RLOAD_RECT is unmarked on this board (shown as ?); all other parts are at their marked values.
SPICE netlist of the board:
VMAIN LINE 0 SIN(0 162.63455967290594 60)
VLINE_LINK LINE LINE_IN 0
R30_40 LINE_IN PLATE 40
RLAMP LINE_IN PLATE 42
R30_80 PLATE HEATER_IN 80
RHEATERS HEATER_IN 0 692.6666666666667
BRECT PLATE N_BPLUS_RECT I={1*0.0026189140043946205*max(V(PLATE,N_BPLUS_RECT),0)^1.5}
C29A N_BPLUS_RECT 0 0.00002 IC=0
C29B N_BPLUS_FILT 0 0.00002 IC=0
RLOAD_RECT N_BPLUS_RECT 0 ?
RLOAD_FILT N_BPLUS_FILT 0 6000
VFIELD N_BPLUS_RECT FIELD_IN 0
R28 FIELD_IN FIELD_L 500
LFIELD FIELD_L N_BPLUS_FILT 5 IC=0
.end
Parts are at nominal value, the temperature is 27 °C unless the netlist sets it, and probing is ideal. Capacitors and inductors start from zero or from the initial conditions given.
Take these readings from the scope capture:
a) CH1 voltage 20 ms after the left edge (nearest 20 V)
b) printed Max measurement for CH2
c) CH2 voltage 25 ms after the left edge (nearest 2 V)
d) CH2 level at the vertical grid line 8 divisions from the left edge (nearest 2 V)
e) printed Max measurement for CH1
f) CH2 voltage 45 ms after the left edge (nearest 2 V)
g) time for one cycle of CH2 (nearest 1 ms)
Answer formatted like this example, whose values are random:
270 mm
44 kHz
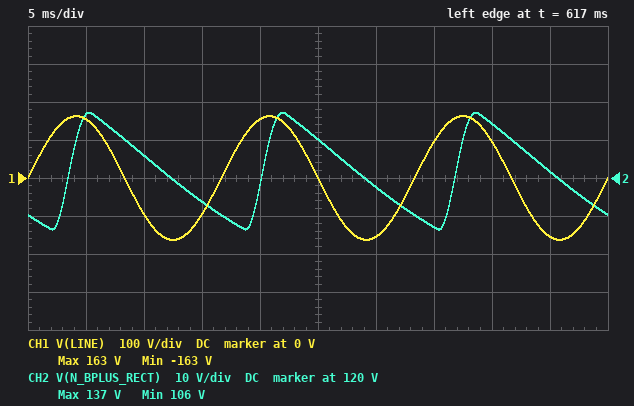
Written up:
160 V
137 V
130 V
134 V
163 V
122 V
17 ms
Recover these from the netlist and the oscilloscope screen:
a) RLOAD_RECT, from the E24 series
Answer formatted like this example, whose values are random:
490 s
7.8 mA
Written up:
4.7 kΩ
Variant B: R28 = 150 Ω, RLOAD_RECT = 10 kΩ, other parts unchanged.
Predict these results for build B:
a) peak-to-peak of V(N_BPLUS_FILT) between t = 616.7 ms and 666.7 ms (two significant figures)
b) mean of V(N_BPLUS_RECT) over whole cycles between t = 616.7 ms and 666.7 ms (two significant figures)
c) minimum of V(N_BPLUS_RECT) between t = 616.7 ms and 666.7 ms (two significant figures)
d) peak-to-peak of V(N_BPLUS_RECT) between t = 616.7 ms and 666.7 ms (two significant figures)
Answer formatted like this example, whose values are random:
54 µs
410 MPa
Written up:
1.4 V
130 V
120 V
24 V
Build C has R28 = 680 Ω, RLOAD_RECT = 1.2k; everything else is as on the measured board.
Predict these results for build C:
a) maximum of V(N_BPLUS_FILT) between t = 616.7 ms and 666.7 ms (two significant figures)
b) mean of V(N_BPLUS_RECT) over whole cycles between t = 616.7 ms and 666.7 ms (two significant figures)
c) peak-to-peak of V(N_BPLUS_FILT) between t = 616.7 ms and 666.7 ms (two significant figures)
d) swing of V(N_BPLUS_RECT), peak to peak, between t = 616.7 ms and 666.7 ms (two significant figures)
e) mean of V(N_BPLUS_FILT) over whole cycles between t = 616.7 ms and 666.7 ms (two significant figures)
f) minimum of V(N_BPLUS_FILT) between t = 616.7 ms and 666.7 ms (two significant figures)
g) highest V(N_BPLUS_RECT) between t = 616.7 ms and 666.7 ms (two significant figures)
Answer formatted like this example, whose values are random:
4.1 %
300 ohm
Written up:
89 V
97 V
3.6 V
61 V
87 V
85 V
130 V
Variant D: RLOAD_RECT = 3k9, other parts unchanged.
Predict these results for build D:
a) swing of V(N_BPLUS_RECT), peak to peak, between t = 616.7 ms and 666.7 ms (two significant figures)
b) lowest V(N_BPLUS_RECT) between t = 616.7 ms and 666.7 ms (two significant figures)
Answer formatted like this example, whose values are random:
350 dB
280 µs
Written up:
34 V
100 V
